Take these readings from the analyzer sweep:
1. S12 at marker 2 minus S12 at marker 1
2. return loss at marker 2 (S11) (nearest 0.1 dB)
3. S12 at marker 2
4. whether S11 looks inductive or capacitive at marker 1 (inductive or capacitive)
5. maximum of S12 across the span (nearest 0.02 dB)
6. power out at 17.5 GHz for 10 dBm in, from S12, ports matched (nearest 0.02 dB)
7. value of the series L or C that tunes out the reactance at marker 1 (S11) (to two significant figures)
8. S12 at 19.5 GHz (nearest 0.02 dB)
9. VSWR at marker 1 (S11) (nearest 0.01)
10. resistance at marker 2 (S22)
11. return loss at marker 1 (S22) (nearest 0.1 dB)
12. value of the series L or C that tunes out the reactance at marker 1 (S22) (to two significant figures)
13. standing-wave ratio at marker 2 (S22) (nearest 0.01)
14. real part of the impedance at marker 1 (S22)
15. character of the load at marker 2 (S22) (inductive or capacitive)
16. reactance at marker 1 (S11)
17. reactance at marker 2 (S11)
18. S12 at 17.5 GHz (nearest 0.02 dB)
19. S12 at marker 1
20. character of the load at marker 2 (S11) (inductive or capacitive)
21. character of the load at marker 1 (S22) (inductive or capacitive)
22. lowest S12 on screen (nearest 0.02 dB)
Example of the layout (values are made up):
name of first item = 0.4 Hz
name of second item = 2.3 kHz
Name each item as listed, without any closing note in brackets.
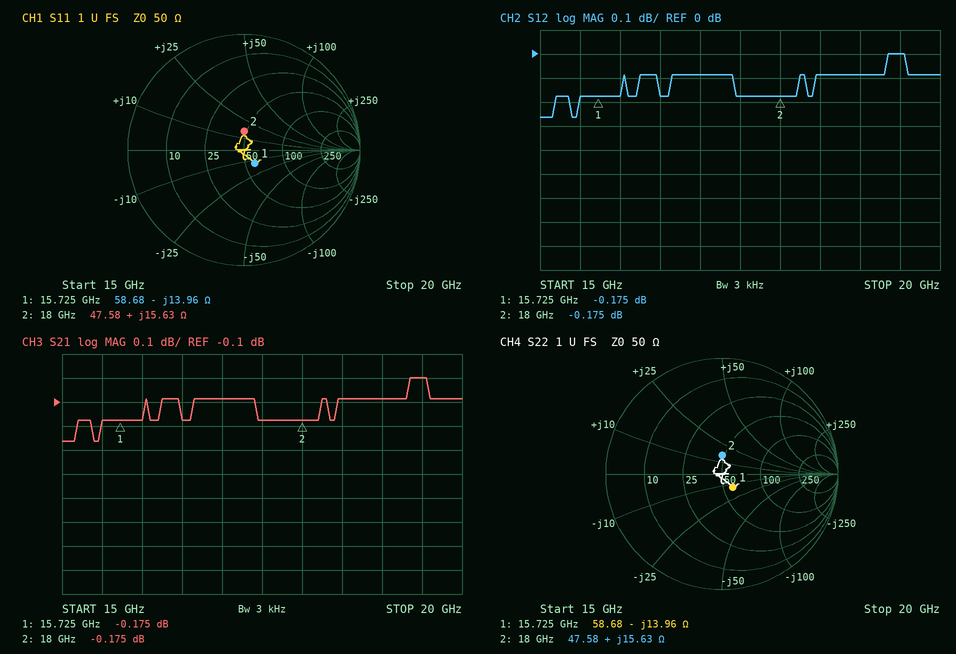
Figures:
S12 at marker 2 minus S12 at marker 1 = 0.000 dB
return loss at marker 2 (S11) = 15.9 dB
S12 at marker 2 = -0.175 dB
whether S11 looks inductive or capacitive at marker 1 = capacitive
maximum of S12 across the span = 0.00 dB
power out at 17.5 GHz for 10 dBm in, from S12, ports matched = 9.82 dBm
value of the series L or C that tunes out the reactance at marker 1 (S11) = 140 pH
S12 at 19.5 GHz = 0.00 dB
VSWR at marker 1 (S11) = 1.35
resistance at marker 2 = 47.58 Ω
return loss at marker 1 (S22) = 16.5 dB
value of the series L or C that tunes out the reactance at marker 1 (S22) = 140 pH
standing-wave ratio at marker 2 (S22) = 1.38
real part of the impedance at marker 1 = 58.68 Ω
character of the load at marker 2 (S22) = inductive
reactance at marker 1 = -13.96 Ω
reactance at marker 2 = +15.63 Ω
S12 at 17.5 GHz = -0.18 dB
S12 at marker 1 = -0.175 dB
character of the load at marker 2 (S11) = inductive
character of the load at marker 1 (S22) = capacitive
lowest S12 on screen = -0.26 dB
